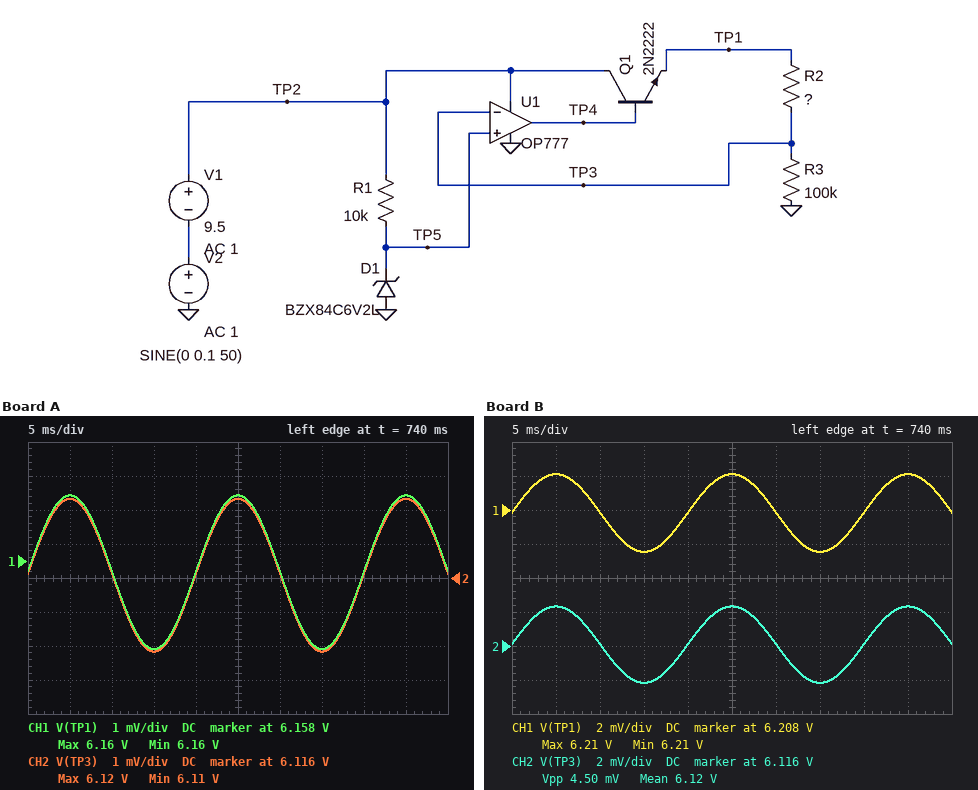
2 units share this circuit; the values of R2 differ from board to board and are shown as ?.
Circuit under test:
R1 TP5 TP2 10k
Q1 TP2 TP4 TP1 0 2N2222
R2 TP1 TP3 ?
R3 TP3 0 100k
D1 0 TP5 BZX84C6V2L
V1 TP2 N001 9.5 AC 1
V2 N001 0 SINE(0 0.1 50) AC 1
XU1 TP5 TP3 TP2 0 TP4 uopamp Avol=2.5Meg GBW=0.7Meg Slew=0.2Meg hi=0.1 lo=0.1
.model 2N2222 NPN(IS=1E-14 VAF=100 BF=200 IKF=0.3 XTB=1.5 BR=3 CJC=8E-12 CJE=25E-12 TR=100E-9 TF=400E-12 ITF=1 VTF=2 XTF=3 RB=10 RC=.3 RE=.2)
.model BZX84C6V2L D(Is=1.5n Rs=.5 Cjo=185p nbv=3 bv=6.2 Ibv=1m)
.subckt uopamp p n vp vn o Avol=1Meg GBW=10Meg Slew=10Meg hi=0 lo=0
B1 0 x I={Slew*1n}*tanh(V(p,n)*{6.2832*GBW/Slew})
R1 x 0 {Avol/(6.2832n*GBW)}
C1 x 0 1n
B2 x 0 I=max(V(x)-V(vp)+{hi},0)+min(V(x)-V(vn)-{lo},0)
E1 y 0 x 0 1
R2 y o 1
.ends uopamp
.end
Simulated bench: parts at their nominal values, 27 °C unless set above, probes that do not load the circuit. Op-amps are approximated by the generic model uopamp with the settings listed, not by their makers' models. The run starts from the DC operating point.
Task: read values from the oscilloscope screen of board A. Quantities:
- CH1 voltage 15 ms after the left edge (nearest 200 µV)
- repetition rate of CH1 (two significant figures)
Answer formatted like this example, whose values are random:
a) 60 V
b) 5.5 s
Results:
a) 6.1554 V
b) 50 Hz
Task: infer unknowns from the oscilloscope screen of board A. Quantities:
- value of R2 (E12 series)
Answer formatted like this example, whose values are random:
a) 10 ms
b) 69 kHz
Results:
a) 680 Ω
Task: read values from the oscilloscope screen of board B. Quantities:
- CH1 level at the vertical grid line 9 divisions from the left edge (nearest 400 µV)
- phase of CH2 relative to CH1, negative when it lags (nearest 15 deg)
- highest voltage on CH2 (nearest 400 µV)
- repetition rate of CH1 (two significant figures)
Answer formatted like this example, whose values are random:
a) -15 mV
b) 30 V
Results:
a) 6.2100 V
b) 0 deg
c) 6.1184 V
d) 50 Hz
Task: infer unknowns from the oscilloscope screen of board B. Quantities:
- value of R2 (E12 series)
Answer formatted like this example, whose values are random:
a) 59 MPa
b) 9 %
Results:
a) 1.5 kΩ
